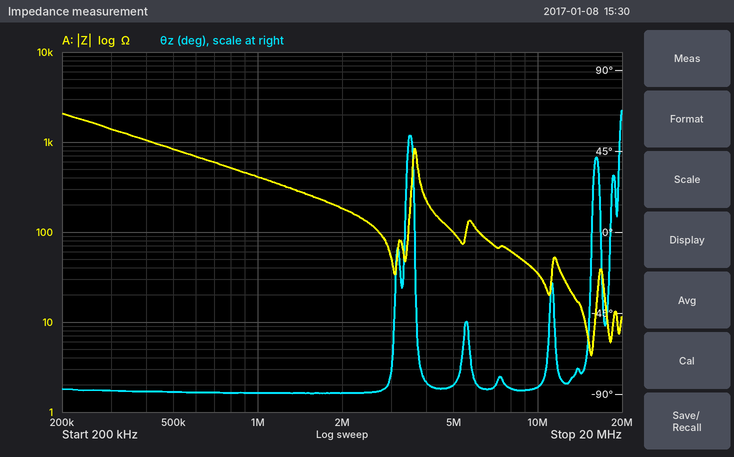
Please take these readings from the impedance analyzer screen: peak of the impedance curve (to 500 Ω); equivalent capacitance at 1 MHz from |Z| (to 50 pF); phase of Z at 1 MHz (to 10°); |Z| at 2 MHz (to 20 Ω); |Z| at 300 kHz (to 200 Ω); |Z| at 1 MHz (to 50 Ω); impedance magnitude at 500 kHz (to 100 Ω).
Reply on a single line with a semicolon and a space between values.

2.0 kΩ; 400 pF; -90°; 180 Ω; 1.4 kΩ; 400 Ω; 800 Ω
